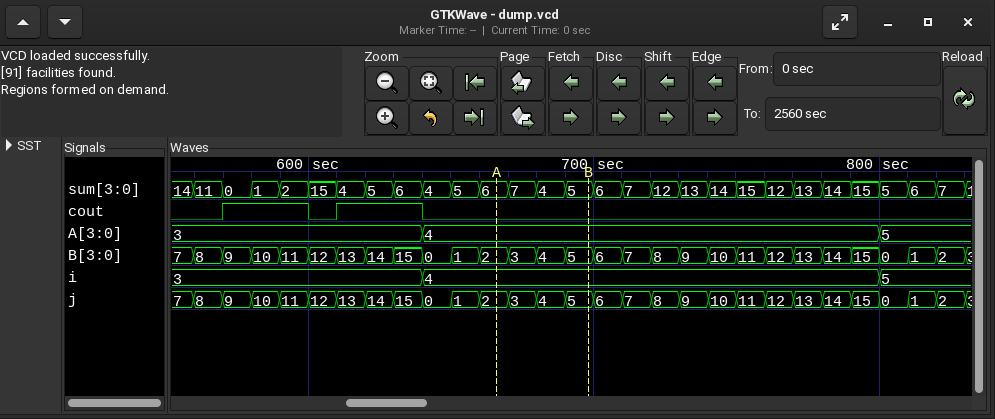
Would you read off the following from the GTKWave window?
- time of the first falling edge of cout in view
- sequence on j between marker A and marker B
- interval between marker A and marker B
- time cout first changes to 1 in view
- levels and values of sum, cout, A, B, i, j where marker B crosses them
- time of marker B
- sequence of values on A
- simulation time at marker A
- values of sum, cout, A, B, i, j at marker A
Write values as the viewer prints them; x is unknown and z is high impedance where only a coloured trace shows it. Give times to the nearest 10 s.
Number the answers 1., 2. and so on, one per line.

1. 600 s
2. 2, 3, 4, 5
3. 30 s
4. 570 s
5. sum=5, cout=0, A=4, B=5, i=4, j=5
6. 700 s
7. 3, 4, 5
8. 670 s
9. sum=6, cout=0, A=4, B=2, i=4, j=2
